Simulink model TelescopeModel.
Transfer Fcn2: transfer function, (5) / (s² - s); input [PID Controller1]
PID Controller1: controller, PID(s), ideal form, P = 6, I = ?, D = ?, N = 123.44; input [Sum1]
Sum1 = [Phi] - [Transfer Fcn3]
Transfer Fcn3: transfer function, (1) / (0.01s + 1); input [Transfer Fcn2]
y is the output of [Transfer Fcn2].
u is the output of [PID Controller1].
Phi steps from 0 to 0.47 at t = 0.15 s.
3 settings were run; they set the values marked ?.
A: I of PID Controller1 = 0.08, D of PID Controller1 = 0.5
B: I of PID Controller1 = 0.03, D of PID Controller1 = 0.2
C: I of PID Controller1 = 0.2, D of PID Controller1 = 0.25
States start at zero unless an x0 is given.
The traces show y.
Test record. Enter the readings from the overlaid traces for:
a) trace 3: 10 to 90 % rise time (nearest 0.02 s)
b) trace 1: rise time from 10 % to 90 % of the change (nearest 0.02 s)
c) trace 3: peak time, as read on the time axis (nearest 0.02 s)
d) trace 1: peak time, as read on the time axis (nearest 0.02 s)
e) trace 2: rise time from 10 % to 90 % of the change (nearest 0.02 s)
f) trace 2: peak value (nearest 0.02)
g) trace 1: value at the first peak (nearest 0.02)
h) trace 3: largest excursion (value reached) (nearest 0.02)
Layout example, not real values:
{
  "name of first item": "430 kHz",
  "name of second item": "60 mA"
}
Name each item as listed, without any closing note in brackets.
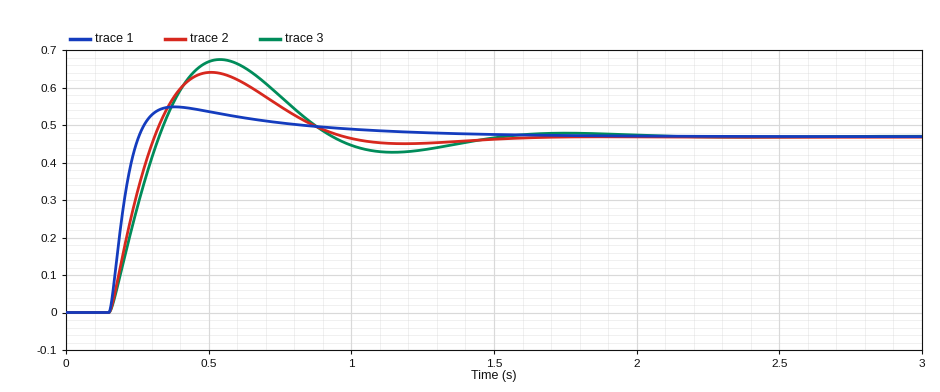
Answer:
{
  "trace 3: 10 to 90 % rise time": "0.14 s",
  "trace 1: rise time from 10 % to 90 % of the change": "0.08 s",
  "trace 3: peak time, as read on the time axis": "0.54 s",
  "trace 1: peak time, as read on the time axis": "0.38 s",
  "trace 2: rise time from 10 % to 90 % of the change": "0.12 s",
  "trace 2: peak value": "0.64",
  "trace 1: value at the first peak": "0.54",
  "trace 3: largest excursion (value reached)": "0.68"
}
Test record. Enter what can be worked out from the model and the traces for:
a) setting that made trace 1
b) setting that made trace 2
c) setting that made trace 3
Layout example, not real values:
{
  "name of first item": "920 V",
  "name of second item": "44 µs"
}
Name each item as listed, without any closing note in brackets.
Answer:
{
  "setting that made trace 1": "A",
  "setting that made trace 2": "C",
  "setting that made trace 3": "B"
}
